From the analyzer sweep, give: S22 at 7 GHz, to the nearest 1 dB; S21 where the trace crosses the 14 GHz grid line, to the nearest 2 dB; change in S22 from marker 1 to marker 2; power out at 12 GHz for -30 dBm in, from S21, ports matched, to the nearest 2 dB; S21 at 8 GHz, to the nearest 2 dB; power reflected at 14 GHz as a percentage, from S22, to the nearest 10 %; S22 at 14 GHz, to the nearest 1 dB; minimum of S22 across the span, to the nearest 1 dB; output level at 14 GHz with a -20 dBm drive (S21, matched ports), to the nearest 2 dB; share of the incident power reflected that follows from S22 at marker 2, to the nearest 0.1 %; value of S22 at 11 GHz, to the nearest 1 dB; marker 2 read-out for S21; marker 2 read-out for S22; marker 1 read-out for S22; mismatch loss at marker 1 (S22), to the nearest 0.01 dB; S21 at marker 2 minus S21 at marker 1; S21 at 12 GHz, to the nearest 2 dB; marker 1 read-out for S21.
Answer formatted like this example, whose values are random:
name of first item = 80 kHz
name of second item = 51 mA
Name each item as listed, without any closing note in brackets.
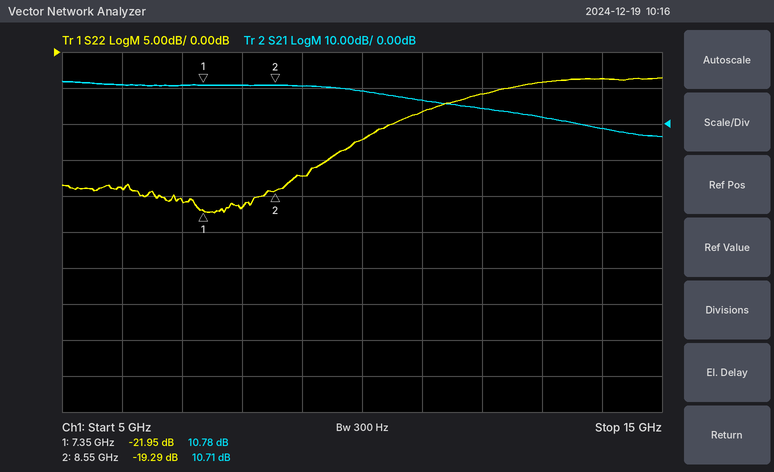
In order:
S22 at 7 GHz, to the nearest 1 dB = -21 dB
S21 where the trace crosses the 14 GHz grid line, to the nearest 2 dB = -2 dB
change in S22 from marker 1 to marker 2 = 2.66 dB
power out at 12 GHz for -30 dBm in, from S21, ports matched, to the nearest 2 dB = -26 dBm
S21 at 8 GHz, to the nearest 2 dB = 10 dB
power reflected at 14 GHz as a percentage, from S22, to the nearest 10 % = 40 %
S22 at 14 GHz, to the nearest 1 dB = -4 dB
minimum of S22 across the span, to the nearest 1 dB = -22 dB
output level at 14 GHz with a -20 dBm drive (S21, matched ports), to the nearest 2 dB = -22 dBm
share of the incident power reflected that follows from S22 at marker 2, to the nearest 0.1 % = 1.2 %
value of S22 at 11 GHz, to the nearest 1 dB = -8 dB
marker 2 read-out for S21 = 10.71 dB
marker 2 read-out for S22 = -19.29 dB
marker 1 read-out for S22 = -21.95 dB
mismatch loss at marker 1 (S22), to the nearest 0.01 dB = 0.03 dB
S21 at marker 2 minus S21 at marker 1 = -0.07 dB
S21 at 12 GHz, to the nearest 2 dB = 4 dB
marker 1 read-out for S21 = 10.78 dB
